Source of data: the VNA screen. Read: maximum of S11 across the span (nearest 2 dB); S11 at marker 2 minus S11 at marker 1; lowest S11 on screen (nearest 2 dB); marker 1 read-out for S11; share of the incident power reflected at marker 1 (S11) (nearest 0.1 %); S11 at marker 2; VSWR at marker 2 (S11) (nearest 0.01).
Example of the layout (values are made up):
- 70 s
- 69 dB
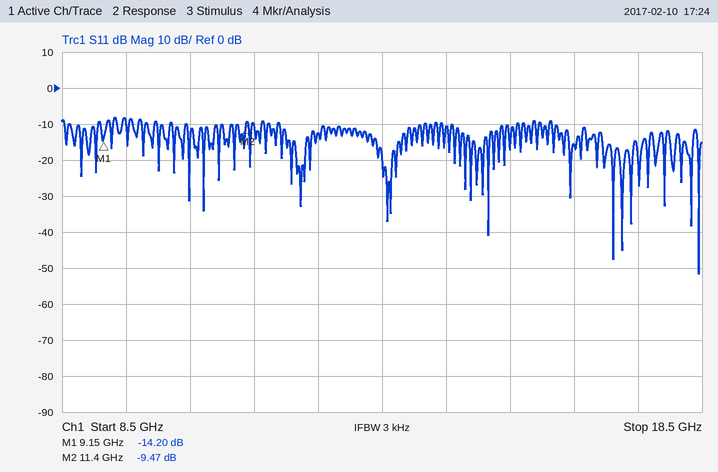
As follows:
- -8 dB
- 4.73 dB
- -52 dB
- -14.20 dB
- 3.8 %
- -9.47 dB
- 2.01
